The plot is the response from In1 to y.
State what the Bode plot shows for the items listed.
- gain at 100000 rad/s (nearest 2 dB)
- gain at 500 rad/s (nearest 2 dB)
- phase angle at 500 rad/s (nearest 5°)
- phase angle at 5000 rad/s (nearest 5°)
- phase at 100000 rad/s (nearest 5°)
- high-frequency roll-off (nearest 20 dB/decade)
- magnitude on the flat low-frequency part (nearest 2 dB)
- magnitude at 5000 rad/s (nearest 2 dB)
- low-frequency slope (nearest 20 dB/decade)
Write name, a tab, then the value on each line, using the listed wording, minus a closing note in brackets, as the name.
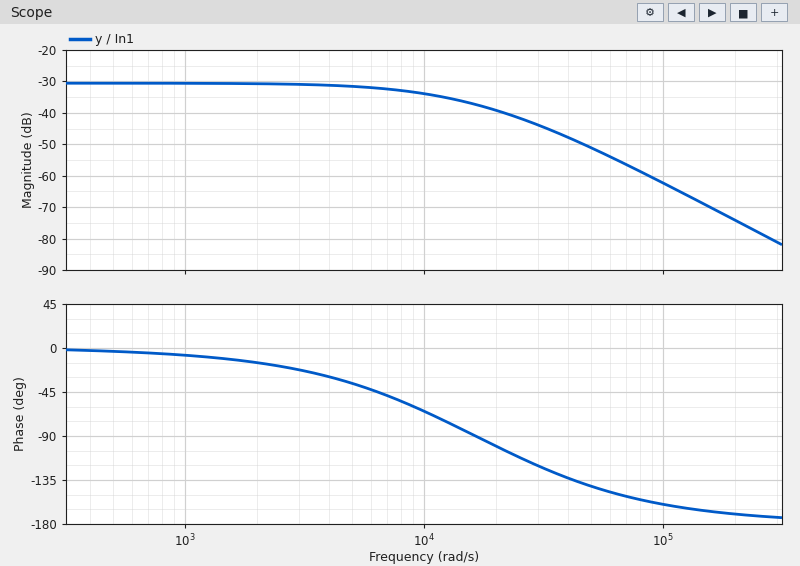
gain at 100000 rad/s	-62 dB
gain at 500 rad/s	-30 dB
phase angle at 500 rad/s	-5°
phase angle at 5000 rad/s	-35°
phase at 100000 rad/s	-160°
high-frequency roll-off	-40 dB/decade
magnitude on the flat low-frequency part	-30 dB
magnitude at 5000 rad/s	-32 dB
low-frequency slope	0 dB/decade
